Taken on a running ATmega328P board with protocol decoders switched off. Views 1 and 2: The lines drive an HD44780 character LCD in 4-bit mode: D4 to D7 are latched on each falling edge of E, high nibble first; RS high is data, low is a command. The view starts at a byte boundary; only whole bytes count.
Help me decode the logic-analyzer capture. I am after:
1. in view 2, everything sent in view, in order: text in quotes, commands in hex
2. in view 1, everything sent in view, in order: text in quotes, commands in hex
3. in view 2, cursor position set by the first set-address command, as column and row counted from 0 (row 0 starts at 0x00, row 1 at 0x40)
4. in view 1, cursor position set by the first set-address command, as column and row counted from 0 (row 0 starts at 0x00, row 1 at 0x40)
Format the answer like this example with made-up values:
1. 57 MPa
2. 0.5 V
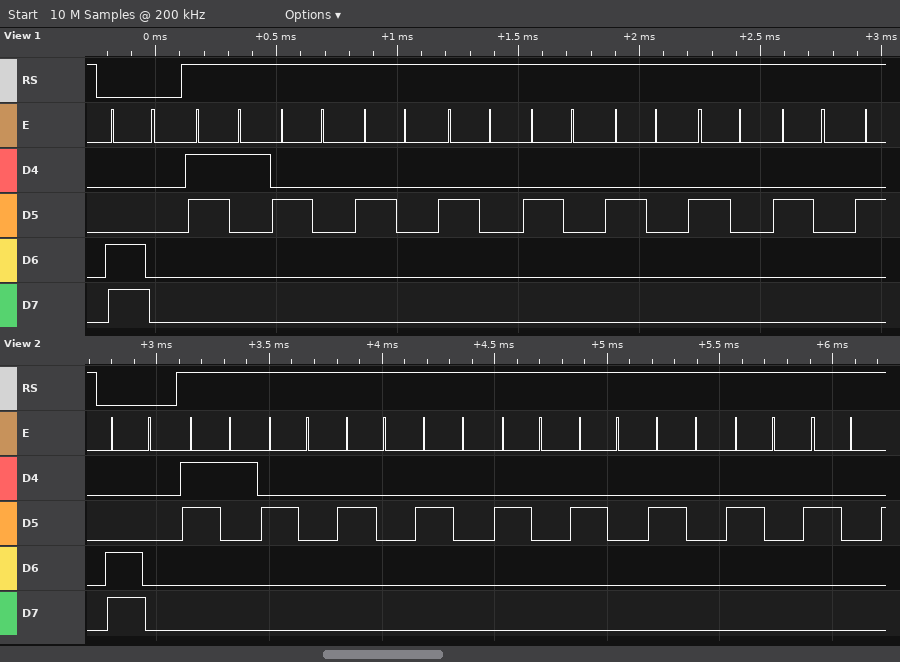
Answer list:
1. 0xC0 "1        "
2. 0xC0 "1       "
3. column 0, row 1
4. column 0, row 1
